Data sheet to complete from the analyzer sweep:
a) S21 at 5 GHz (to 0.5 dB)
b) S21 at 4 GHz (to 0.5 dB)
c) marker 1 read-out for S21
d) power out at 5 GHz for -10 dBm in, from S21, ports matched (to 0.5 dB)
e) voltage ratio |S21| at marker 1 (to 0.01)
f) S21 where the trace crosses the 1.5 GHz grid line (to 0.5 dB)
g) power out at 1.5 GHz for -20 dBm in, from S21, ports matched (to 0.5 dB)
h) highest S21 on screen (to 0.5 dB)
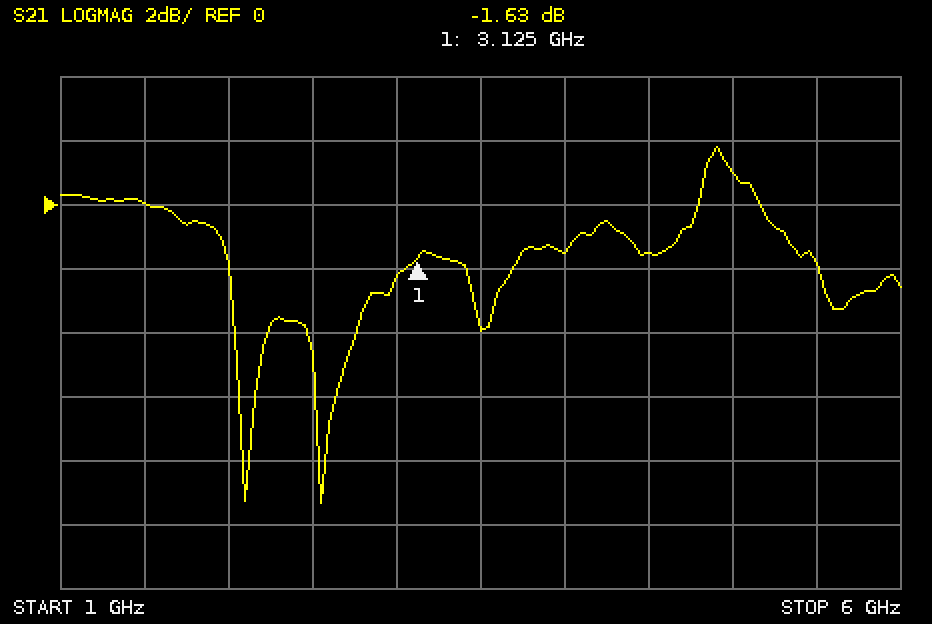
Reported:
1.0 dB
-1.5 dB
-1.63 dB
-9.0 dBm
0.83
0.0 dB
-20.0 dBm
2.0 dB
